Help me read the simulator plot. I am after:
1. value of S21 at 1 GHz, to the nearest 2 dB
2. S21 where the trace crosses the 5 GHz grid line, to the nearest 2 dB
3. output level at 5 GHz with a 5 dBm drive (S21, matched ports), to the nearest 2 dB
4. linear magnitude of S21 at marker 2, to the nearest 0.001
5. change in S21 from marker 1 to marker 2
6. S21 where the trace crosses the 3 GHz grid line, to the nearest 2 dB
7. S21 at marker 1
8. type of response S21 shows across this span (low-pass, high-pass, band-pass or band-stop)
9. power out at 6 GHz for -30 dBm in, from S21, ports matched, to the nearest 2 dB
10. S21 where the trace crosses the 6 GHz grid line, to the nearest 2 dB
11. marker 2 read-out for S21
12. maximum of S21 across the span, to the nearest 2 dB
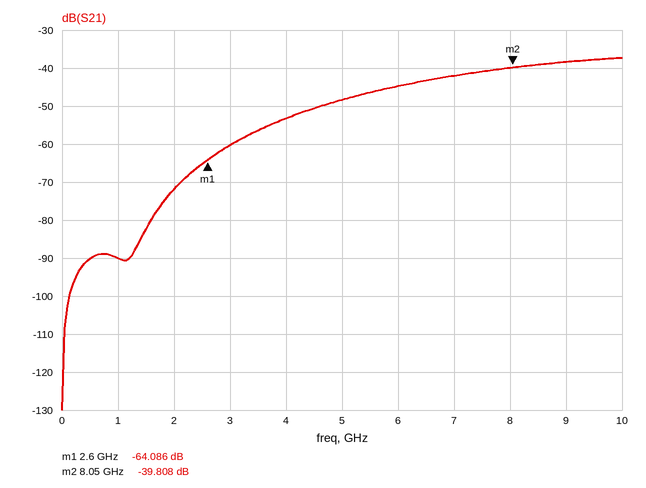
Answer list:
-90 dB
-48 dB
-44 dBm
0.010
24.278 dB
-60 dB
-64.086 dB
high-pass
-74 dBm
-44 dB
-39.808 dB
-38 dB
